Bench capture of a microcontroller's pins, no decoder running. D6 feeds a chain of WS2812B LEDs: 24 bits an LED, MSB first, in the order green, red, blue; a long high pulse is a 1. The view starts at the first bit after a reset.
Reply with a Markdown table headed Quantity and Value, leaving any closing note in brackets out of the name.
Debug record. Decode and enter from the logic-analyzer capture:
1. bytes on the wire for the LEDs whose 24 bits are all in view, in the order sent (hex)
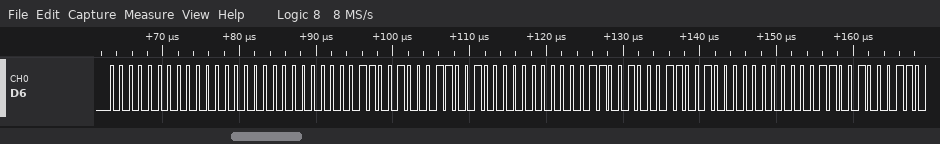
| Quantity | Value |
|---|---|
| bytes on the wire for the LEDs whose 24 bits are all in view, in the order sent | 00 00 00 32 32 00 32 32 00 |
